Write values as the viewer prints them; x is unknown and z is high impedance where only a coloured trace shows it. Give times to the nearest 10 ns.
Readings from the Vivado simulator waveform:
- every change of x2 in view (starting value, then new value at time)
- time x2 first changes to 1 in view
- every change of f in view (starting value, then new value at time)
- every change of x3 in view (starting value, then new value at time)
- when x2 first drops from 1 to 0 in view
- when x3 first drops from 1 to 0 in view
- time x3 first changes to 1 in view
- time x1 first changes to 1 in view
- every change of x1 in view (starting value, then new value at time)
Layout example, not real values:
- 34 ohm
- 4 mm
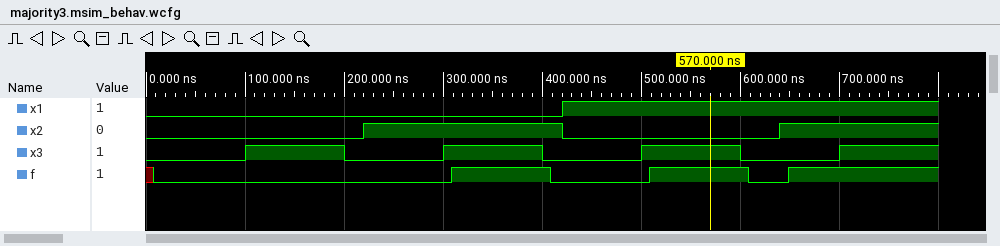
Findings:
- 0, 1 at 220 ns, 0 at 420 ns, 1 at 640 ns
- 220 ns
- x, 0 at 10 ns, 1 at 310 ns, 0 at 410 ns, 1 at 510 ns, 0 at 610 ns, 1 at 650 ns
- 0, 1 at 100 ns, 0 at 200 ns, 1 at 300 ns, 0 at 400 ns, 1 at 500 ns, 0 at 600 ns, 1 at 700 ns
- 420 ns
- 200 ns
- 100 ns
- 420 ns
- 0, 1 at 420 ns
